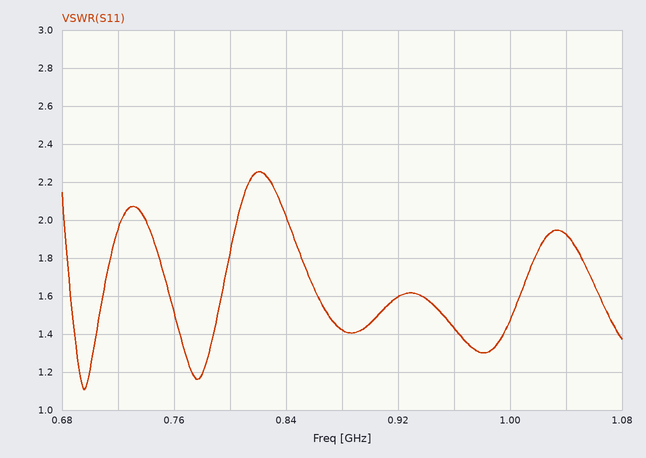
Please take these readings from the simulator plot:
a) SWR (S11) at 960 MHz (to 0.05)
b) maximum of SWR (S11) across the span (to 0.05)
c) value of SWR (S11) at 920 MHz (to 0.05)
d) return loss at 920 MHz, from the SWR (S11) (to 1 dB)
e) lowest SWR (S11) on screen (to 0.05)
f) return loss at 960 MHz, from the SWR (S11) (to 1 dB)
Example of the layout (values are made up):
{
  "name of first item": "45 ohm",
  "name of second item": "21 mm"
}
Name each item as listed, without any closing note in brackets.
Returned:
{
  "SWR (S11) at 960 MHz": "1.45",
  "maximum of SWR (S11) across the span": "2.25",
  "value of SWR (S11) at 920 MHz": "1.60",
  "return loss at 920 MHz, from the SWR (S11)": "13 dB",
  "lowest SWR (S11) on screen": "1.10",
  "return loss at 960 MHz, from the SWR (S11)": "15 dB"
}
